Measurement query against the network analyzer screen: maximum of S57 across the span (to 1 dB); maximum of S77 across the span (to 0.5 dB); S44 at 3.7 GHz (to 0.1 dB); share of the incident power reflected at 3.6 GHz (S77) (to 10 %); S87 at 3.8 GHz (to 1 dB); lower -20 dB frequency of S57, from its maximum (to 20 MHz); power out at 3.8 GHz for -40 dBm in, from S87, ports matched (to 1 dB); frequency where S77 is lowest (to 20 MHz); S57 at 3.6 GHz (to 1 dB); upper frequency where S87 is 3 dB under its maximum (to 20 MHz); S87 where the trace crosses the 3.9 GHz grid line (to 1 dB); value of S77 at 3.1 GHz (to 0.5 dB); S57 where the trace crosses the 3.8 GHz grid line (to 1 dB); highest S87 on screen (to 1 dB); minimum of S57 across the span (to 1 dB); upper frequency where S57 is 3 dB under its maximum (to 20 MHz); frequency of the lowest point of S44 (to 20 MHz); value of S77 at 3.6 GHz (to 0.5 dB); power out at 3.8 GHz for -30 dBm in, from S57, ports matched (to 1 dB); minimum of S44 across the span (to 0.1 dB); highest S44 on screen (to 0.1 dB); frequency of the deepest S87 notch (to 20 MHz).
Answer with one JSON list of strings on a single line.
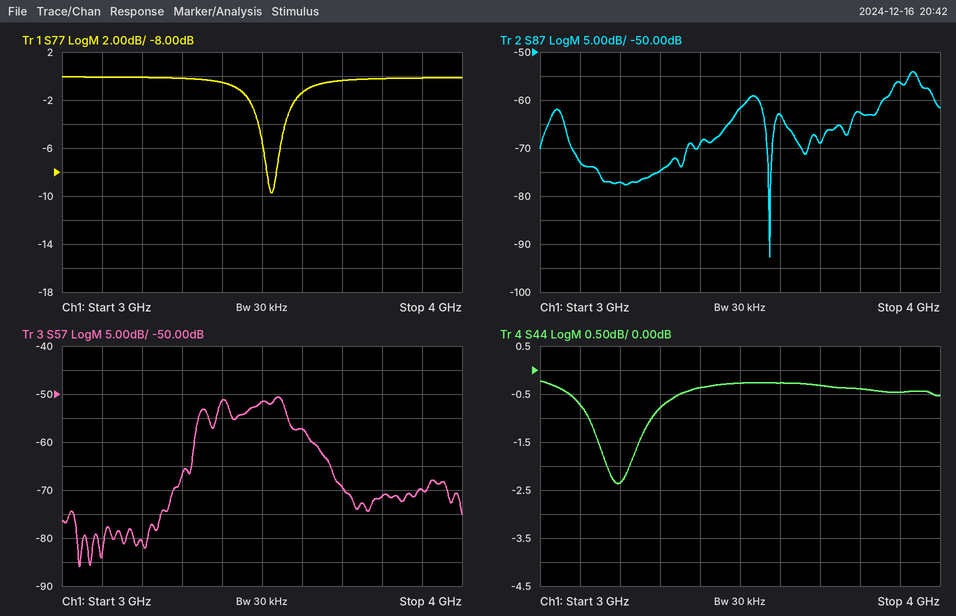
["-51 dB", "0.0 dB", "-0.3 dB", "70 %", "-63 dB", "3.28 GHz", "-103 dBm", "3.52 GHz", "-57 dB", "3.96 GHz", "-56 dB", "0.0 dB", "-71 dB", "-54 dB", "-86 dB", "3.56 GHz", "3.20 GHz", "-1.5 dB", "-101 dBm", "-2.4 dB", "-0.2 dB", "3.58 GHz"]
